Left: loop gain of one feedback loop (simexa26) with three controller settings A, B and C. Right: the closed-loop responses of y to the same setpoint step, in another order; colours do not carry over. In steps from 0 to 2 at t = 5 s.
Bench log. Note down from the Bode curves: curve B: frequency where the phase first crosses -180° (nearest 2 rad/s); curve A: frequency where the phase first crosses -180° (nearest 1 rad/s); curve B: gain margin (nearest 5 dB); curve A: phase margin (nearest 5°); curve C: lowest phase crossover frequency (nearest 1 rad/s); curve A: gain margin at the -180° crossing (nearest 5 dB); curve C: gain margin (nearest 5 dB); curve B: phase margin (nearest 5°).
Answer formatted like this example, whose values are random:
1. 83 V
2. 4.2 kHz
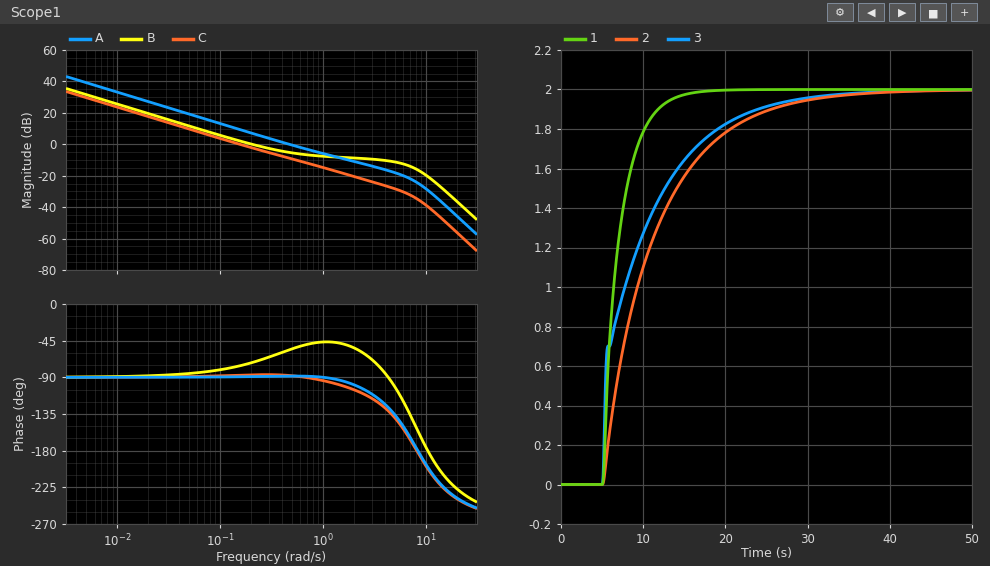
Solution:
1. 10 rad/s
2. 8 rad/s
3. 20 dB
4. 90°
5. 8 rad/s
6. 25 dB
7. 35 dB
8. 110°
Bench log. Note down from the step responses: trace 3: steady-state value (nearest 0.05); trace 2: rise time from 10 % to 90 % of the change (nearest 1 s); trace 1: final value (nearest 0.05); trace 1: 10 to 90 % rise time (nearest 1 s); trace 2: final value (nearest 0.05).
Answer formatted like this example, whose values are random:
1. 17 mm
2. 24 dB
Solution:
1. 2.00
2. 15 s
3. 2.00
4. 5 s
5. 2.00
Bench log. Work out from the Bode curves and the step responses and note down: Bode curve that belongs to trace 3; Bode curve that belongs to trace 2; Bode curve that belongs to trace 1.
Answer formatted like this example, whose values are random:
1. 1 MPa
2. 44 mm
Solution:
1. B
2. C
3. A
